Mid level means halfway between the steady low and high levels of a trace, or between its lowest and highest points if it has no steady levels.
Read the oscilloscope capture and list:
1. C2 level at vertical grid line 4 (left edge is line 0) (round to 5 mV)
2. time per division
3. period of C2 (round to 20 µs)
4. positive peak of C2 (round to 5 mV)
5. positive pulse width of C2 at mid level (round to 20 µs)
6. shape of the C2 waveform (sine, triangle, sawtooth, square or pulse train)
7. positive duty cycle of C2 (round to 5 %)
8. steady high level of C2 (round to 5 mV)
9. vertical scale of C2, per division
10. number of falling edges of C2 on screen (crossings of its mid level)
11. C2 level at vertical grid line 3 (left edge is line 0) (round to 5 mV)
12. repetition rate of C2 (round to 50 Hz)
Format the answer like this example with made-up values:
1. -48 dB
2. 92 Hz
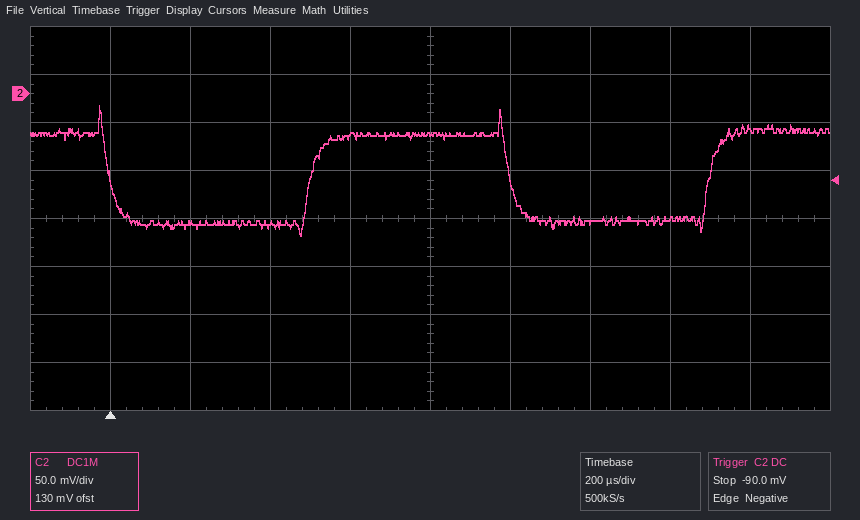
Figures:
1. -45 mV
2. 200 µs
3. 1.00 ms
4. -10 mV
5. 500 µs
6. square
7. 50 %
8. -40 mV
9. 50 mV
10. 2
11. -135 mV
12. 1.00 kHz
